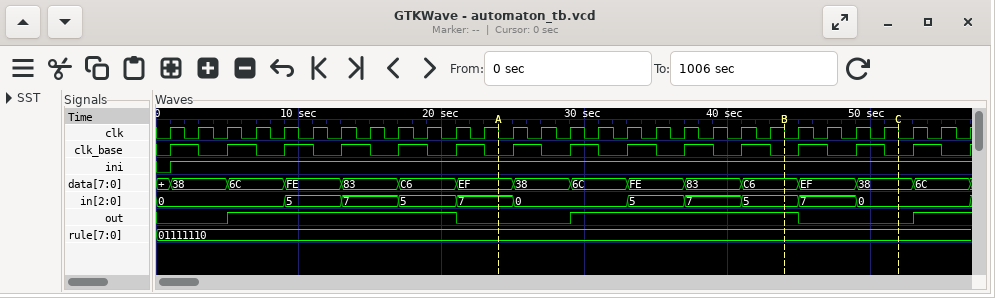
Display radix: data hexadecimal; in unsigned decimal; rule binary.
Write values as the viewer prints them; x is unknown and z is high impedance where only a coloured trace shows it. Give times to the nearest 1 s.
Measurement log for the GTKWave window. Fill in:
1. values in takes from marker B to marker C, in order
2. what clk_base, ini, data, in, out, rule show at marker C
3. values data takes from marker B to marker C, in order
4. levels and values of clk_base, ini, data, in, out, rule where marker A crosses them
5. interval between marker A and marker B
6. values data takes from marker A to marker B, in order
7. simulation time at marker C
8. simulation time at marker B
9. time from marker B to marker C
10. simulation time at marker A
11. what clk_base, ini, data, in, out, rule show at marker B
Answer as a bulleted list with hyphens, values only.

- 5, 7, 0
- clk_base=0, ini=1, data=38, in=0, out=0, rule=01111110
- C6, EF, 38
- clk_base=0, ini=1, data=EF, in=7, out=0, rule=01111110
- 20 s
- EF, 38, 6C, FE, 83, C6
- 52 s
- 44 s
- 8 s
- 24 s
- clk_base=0, ini=1, data=C6, in=5, out=1, rule=01111110
